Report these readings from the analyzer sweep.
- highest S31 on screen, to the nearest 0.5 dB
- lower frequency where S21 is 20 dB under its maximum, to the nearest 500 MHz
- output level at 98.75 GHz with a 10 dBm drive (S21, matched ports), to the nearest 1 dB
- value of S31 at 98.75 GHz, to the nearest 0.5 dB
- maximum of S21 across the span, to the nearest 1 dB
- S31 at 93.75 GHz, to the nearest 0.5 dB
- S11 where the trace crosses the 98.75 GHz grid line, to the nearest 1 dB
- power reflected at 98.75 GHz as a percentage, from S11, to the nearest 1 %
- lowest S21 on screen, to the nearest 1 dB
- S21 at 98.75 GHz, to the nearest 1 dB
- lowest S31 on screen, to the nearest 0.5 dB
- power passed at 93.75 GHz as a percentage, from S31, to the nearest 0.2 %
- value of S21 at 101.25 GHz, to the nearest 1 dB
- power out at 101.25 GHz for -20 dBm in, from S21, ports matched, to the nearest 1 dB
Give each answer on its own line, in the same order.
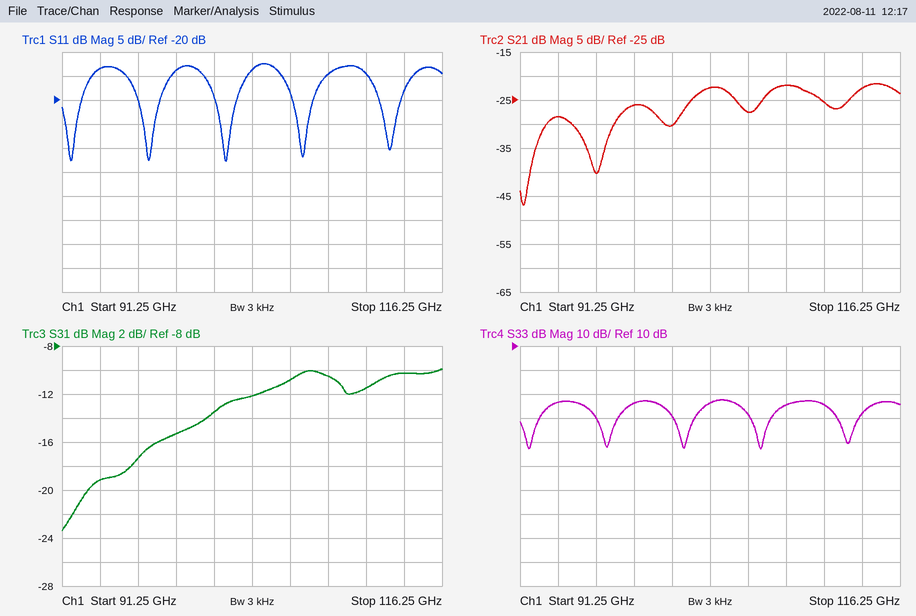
-10.0 dB
92.0 GHz
-16 dBm
-15.5 dB
-22 dB
-19.0 dB
-14 dB
4 %
-47 dB
-26 dB
-23.5 dB
1.2 %
-30 dB
-50 dBm
